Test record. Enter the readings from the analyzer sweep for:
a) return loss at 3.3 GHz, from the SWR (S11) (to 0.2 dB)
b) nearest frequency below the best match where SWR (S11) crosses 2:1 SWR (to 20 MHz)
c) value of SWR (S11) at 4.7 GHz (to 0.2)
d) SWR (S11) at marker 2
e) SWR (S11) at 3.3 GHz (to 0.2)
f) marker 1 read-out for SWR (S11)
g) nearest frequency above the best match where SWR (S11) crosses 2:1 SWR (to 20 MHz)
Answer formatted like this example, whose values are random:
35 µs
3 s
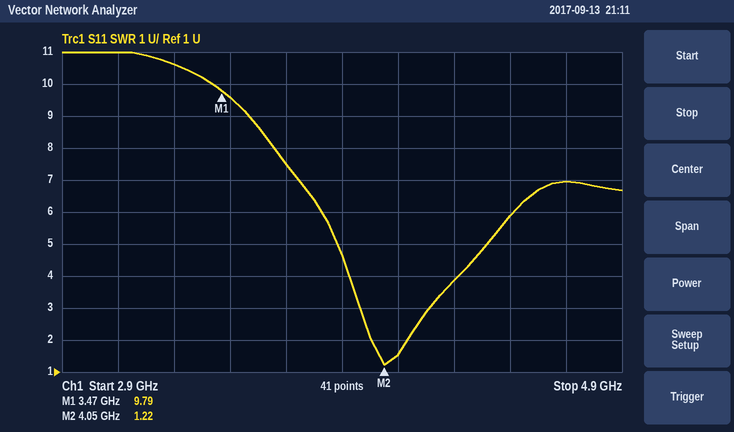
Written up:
1.6 dB
4.00 GHz
7.0
1.22
10.6
9.79
4.14 GHz
